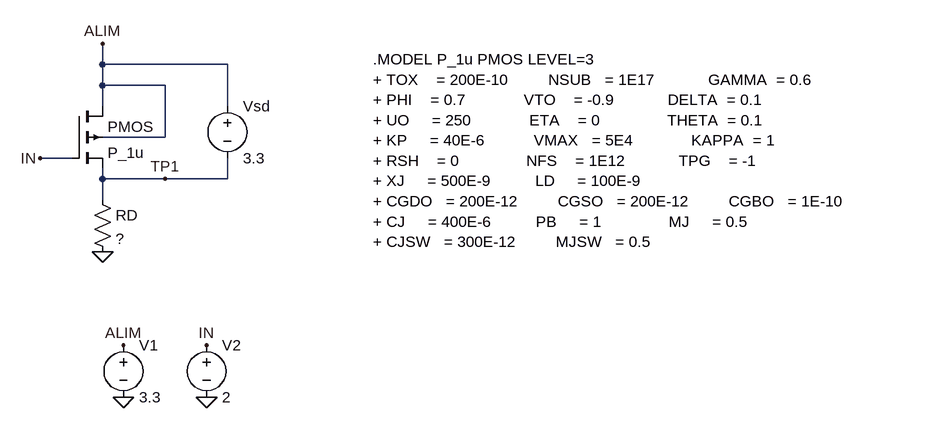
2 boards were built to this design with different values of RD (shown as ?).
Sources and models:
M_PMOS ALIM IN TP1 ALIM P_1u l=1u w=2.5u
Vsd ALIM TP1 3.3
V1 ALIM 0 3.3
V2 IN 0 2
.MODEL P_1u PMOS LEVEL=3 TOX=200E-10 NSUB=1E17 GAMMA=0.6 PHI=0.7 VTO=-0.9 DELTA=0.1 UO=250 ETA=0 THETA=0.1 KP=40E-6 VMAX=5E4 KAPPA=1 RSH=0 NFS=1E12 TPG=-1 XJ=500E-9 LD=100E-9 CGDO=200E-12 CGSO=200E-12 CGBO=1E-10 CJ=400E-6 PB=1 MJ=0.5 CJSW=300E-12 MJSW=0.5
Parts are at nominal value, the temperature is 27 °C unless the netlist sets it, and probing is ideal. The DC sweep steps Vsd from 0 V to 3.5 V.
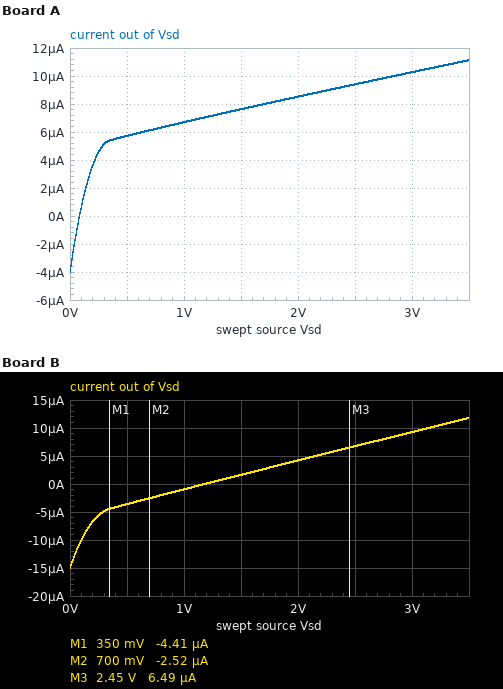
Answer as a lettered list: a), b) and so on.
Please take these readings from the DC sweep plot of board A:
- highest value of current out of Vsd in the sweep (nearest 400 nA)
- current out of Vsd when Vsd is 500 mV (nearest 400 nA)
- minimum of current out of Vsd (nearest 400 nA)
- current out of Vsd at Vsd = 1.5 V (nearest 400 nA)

a) 11.2 µA
b) 5.6 µA
c) -4.0 µA
d) 7.6 µA
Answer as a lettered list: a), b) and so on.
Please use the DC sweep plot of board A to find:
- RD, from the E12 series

a) 820 kΩ
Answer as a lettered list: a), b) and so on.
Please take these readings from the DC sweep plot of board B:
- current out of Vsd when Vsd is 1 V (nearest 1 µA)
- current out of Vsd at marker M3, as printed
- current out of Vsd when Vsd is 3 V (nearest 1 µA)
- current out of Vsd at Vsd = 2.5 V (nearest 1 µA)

a) -1 µA
b) 6.49 µA
c) 9 µA
d) 7 µA
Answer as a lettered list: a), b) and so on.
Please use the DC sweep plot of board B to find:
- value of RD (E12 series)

a) 220 kΩ
